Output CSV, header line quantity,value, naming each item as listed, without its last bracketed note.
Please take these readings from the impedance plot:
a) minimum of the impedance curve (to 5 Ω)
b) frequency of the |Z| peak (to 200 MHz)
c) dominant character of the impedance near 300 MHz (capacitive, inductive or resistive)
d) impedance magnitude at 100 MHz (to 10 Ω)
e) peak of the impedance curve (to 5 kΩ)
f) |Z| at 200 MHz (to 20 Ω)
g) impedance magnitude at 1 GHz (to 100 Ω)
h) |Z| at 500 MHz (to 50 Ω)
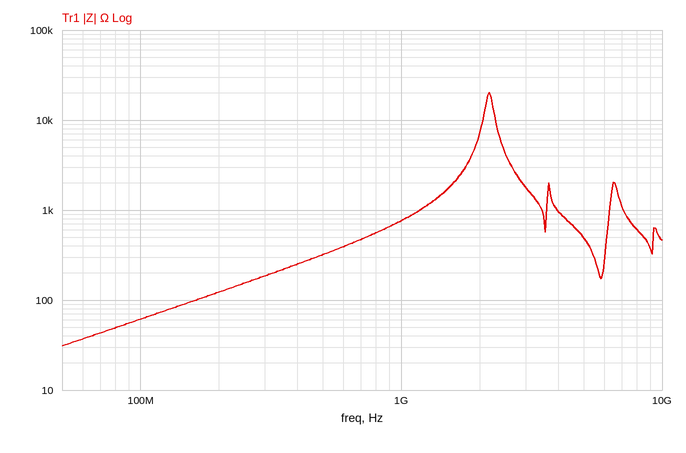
quantity,value
minimum of the impedance curve,30 Ω
frequency of the |Z| peak,2.2 GHz
dominant character of the impedance near 300 MHz,inductive
impedance magnitude at 100 MHz,60 Ω
peak of the impedance curve,20 kΩ
|Z| at 200 MHz,120 Ω
impedance magnitude at 1 GHz,800 Ω
|Z| at 500 MHz,300 Ω
